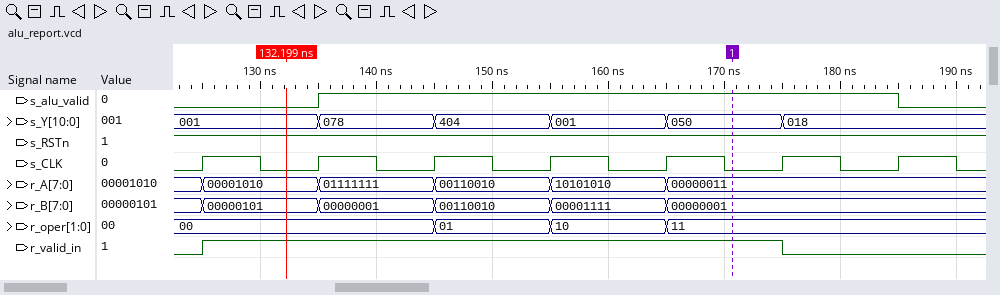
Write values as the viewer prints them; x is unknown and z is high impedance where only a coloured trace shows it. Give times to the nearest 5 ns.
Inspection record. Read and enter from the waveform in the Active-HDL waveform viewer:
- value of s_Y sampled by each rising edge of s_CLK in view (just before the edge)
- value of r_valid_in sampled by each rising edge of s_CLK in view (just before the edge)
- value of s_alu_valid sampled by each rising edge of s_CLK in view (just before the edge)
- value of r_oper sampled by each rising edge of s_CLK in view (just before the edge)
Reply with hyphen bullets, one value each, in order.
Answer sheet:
- 001, 001, 078, 404, 001, 050, 018
- 0 1 1 1 1 1 0
- 0 0 1 1 1 1 1
- 00, 00, 00, 01, 10, 11, 11
